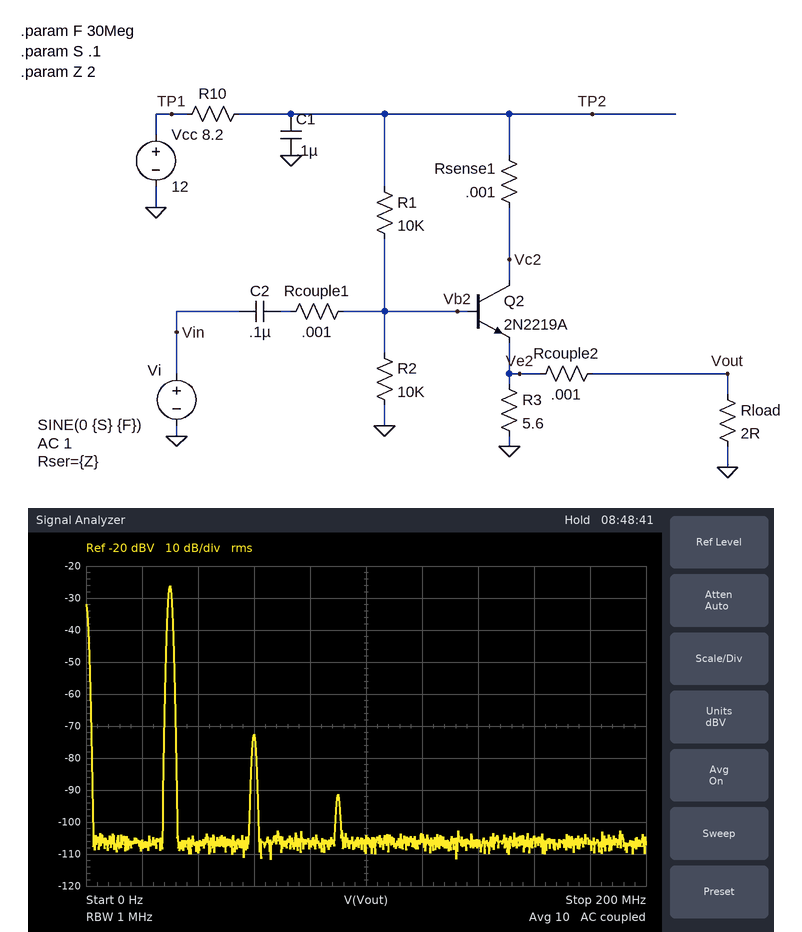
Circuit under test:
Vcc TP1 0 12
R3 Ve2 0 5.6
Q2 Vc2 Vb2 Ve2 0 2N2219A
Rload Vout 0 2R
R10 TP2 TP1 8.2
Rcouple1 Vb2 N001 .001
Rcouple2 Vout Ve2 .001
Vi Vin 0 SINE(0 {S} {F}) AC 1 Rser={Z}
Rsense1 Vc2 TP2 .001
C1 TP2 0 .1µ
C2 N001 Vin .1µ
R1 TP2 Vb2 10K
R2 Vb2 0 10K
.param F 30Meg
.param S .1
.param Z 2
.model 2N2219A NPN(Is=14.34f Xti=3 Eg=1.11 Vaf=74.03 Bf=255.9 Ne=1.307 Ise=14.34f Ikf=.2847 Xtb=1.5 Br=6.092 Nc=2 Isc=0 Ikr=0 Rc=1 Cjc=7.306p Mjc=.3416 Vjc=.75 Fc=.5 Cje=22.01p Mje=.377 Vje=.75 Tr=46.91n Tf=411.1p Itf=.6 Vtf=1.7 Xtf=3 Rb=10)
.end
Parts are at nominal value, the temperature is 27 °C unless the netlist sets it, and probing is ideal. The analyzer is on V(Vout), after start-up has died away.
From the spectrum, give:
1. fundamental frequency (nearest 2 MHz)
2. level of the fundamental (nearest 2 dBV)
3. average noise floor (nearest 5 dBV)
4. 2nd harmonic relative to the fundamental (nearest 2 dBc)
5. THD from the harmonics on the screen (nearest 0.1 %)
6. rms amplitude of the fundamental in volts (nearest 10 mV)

30 MHz
-26 dBV
-105 dBV
-46 dBc
0.5 %
50 mV
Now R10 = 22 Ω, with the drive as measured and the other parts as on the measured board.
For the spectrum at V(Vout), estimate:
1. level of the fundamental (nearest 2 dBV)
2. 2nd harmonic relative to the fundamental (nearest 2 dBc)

-26 dBV
-44 dBc
